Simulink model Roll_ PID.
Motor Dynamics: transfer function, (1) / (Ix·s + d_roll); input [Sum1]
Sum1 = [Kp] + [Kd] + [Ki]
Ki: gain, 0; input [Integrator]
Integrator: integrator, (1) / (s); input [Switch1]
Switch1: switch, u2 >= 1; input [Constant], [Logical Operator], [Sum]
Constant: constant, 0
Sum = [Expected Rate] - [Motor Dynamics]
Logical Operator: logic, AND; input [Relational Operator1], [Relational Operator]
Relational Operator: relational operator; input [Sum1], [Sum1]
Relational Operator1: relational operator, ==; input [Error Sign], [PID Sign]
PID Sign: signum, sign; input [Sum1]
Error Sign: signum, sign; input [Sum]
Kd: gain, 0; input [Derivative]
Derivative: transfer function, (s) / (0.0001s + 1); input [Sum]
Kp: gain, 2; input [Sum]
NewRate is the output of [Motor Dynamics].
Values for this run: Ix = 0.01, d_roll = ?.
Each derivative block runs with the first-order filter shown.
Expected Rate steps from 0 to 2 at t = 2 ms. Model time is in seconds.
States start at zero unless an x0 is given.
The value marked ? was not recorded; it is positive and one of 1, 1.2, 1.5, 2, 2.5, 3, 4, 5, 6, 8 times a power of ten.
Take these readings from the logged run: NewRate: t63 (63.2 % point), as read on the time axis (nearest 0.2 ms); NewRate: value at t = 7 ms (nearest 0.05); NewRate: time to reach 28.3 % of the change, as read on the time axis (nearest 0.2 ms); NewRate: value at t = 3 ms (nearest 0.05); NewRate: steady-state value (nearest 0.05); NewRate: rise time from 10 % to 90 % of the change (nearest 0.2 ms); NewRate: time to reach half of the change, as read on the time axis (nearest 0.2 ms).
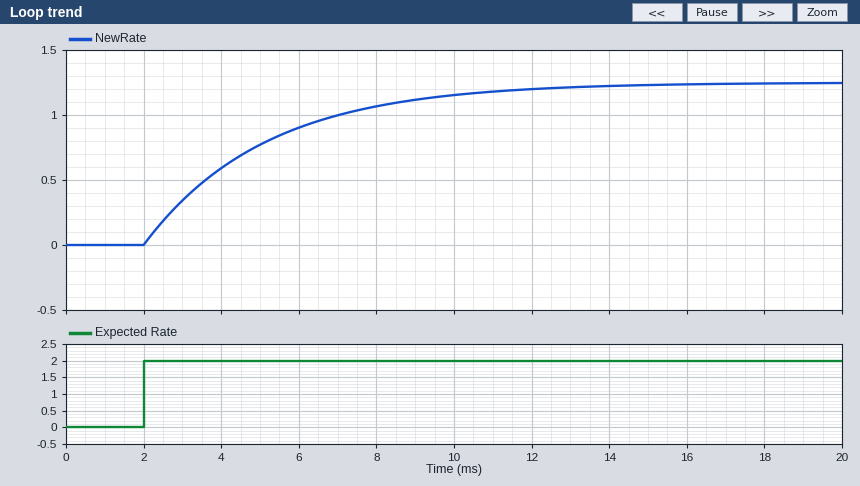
5.2 ms
1.00
3.0 ms
0.35
1.25
6.8 ms
4.2 ms
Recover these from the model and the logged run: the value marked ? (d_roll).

1.2
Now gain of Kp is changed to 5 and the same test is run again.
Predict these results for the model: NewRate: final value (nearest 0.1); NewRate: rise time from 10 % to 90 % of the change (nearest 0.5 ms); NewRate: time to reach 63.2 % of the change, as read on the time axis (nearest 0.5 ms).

1.6
3.5 ms
3.5 ms
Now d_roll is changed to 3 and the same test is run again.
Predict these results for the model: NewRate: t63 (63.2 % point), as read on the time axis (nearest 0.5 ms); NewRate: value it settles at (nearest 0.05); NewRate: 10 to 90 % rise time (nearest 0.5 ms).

4.0 ms
0.80
4.5 ms
